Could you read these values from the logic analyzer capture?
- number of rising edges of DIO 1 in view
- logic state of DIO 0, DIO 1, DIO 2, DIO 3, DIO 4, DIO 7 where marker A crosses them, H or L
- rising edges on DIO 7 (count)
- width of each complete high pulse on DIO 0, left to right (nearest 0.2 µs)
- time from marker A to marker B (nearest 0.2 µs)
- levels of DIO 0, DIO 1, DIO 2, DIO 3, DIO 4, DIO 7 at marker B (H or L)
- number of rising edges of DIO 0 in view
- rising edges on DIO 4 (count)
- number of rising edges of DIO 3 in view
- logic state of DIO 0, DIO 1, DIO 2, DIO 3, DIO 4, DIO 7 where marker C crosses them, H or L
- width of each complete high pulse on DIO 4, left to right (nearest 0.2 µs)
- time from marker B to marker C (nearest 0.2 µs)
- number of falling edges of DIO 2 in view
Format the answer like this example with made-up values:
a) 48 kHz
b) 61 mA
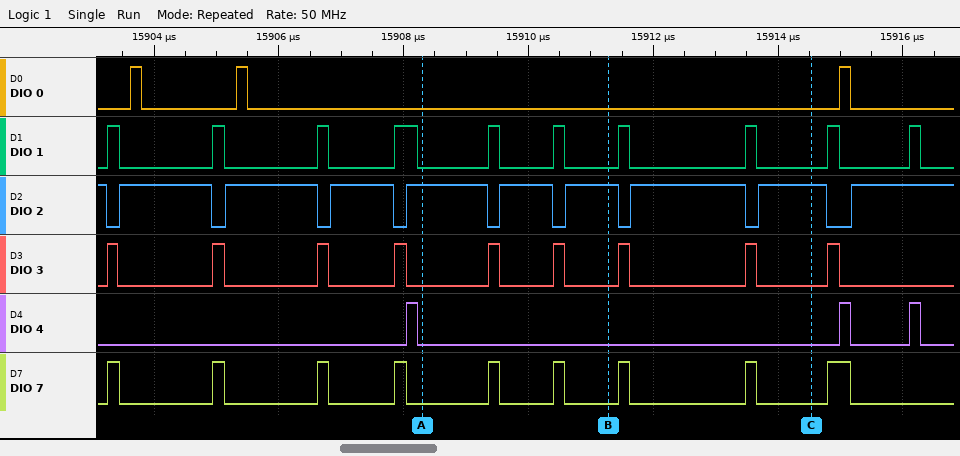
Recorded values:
a) 10
b) DIO 0=L, DIO 1=L, DIO 2=H, DIO 3=L, DIO 4=L, DIO 7=L
c) 9
d) 0.2 µs, 0.2 µs, 0.2 µs
e) 3 µs
f) DIO 0=L, DIO 1=L, DIO 2=H, DIO 3=L, DIO 4=L, DIO 7=L
g) 3
h) 3
i) 9
j) DIO 0=L, DIO 1=L, DIO 2=H, DIO 3=L, DIO 4=L, DIO 7=L
k) 0.2 µs, 0.2 µs, 0.2 µs
l) 3.2 µs
m) 9
